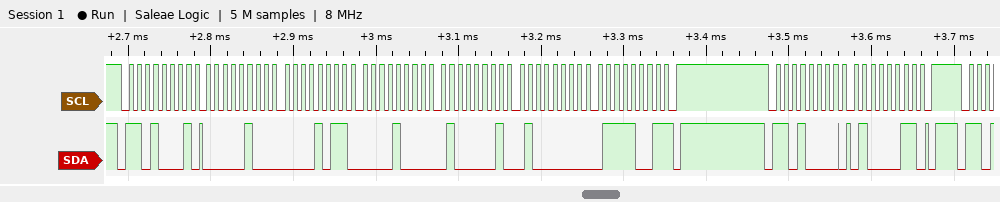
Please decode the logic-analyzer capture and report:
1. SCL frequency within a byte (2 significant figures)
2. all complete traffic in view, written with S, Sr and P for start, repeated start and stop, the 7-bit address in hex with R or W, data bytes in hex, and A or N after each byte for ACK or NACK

100 kHz
S 68R A 04 A 0B A 08 A 41 A 40 A 79 N P S 68W A 43 A P
